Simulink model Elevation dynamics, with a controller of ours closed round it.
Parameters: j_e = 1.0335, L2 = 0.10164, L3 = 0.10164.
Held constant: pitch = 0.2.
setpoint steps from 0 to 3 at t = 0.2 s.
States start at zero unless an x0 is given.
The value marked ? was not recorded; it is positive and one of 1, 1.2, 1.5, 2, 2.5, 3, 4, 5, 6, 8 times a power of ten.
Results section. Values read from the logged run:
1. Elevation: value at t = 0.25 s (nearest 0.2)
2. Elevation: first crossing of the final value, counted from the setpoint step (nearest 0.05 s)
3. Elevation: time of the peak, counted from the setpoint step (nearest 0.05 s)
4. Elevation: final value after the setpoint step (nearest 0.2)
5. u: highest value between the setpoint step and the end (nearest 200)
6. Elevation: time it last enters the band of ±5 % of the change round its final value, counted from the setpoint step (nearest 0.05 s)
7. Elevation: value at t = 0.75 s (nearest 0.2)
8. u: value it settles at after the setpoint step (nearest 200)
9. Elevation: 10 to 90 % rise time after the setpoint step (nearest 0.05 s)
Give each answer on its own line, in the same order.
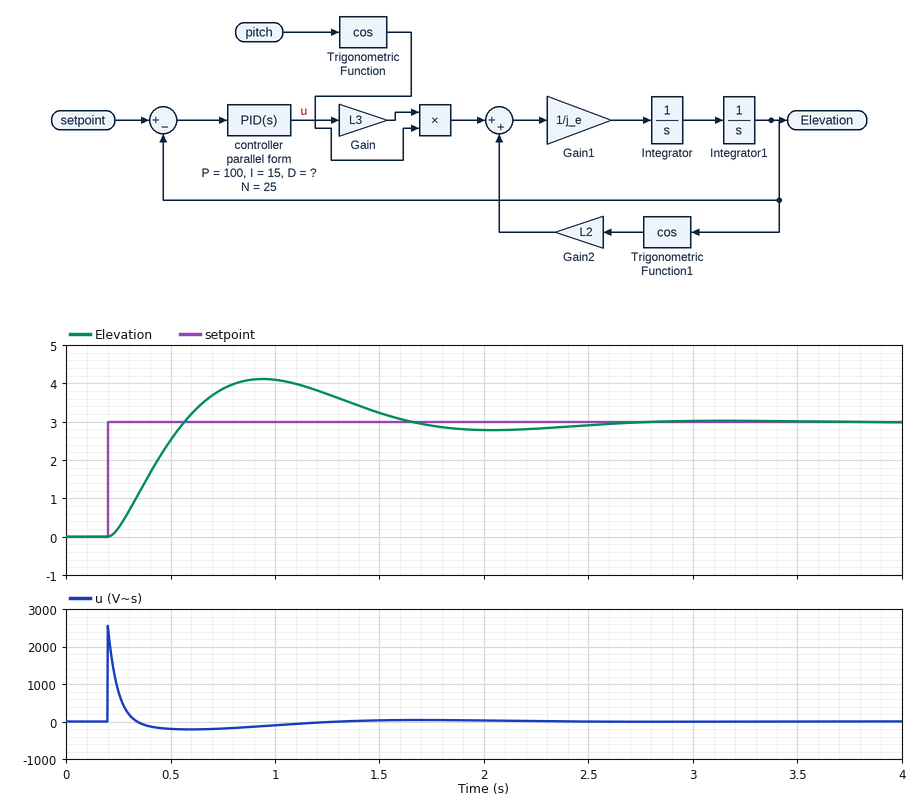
0.2
0.35 s
0.75 s
3.0
2600
2.15 s
3.8
0
0.25 s
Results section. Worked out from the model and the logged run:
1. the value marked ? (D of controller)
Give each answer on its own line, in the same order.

30
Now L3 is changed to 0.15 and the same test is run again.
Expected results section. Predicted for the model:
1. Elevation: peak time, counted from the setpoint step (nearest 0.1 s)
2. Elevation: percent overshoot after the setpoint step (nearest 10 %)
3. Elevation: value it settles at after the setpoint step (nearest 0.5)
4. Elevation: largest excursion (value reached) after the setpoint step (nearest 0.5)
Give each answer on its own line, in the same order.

0.6 s
30 %
3.0
4.0
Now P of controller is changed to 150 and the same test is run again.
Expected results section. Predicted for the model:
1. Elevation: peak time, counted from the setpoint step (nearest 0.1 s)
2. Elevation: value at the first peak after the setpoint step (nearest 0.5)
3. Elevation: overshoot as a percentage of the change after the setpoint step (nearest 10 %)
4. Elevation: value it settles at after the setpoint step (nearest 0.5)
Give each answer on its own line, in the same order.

0.6 s
4.5
40 %
3.0
